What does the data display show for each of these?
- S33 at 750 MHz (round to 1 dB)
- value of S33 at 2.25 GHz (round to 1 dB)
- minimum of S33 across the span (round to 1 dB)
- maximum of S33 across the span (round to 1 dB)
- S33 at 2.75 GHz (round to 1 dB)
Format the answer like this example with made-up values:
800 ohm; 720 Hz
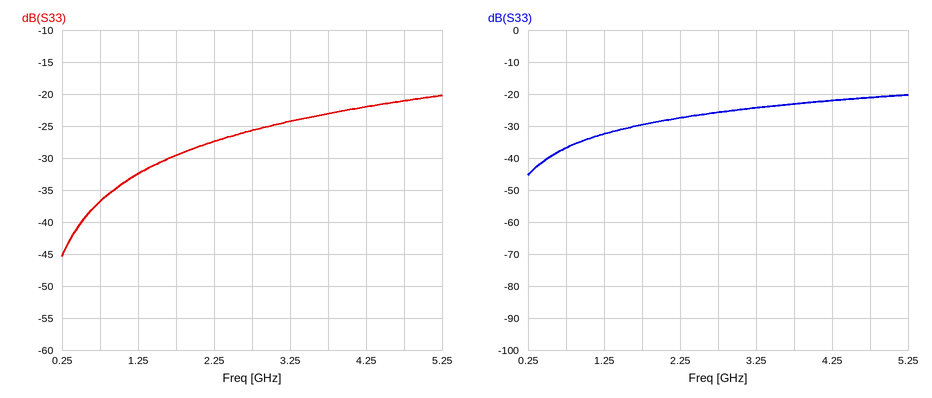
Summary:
-37 dB; -27 dB; -45 dB; -20 dB; -26 dB
